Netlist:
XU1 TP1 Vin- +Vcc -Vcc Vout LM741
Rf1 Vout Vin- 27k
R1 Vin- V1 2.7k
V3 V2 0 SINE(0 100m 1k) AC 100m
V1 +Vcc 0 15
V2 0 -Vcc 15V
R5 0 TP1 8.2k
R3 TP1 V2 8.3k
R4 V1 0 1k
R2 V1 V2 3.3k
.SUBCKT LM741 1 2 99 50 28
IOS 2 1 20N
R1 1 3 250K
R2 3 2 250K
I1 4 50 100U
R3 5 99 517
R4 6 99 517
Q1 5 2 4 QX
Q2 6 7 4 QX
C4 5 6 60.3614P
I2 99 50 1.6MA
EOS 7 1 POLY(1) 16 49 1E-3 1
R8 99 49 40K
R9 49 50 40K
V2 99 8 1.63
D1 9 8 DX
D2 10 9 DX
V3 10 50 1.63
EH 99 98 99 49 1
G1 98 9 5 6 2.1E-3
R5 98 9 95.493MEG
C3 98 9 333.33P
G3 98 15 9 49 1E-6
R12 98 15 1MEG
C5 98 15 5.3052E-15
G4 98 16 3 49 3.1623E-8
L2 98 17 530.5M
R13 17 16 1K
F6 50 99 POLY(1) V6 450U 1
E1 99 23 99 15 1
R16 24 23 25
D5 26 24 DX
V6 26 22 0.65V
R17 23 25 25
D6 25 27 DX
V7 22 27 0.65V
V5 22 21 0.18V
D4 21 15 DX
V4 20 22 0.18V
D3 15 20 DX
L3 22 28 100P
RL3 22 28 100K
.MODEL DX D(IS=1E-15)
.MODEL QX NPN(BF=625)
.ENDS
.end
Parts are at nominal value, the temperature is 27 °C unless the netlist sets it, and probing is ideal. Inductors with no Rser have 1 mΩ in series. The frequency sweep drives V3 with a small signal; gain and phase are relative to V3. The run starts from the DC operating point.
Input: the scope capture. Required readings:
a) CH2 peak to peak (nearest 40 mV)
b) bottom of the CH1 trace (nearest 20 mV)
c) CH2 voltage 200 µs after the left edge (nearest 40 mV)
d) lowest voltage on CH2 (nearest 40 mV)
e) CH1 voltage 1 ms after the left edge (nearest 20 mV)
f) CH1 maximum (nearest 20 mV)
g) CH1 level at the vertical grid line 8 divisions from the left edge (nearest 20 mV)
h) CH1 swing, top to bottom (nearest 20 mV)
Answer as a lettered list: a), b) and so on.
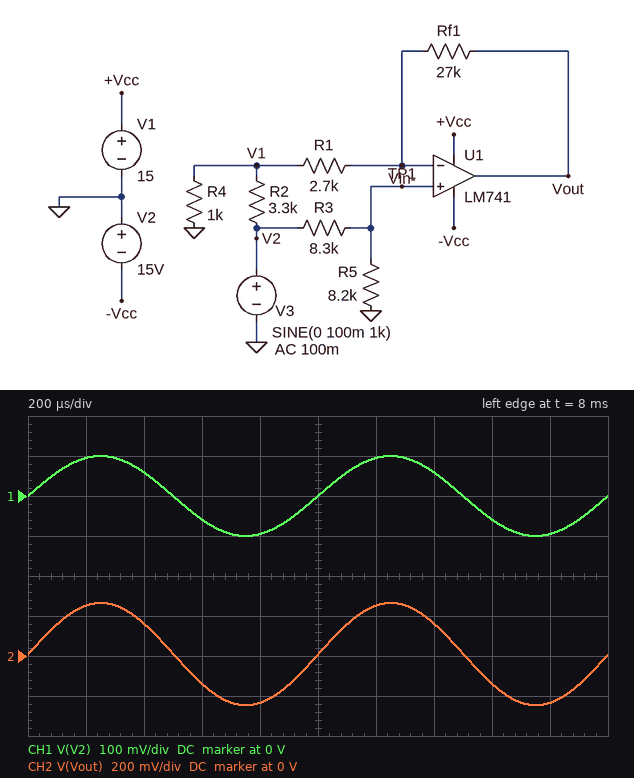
a) 520 mV
b) -100 mV
c) 240 mV
d) -240 mV
e) 0 V
f) 100 mV
g) -60 mV
h) 200 mV
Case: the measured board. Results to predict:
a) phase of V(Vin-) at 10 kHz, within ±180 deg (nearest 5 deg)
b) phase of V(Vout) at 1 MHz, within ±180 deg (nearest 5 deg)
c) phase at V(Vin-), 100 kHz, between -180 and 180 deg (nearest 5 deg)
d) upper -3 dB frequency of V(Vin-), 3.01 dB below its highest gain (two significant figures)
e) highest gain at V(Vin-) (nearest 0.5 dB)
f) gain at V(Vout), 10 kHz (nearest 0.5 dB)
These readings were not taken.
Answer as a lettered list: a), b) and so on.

a) -5 deg
b) -100 deg
c) -20 deg
d) 140 kHz
e) -6.0 dB
f) 8.0 dB
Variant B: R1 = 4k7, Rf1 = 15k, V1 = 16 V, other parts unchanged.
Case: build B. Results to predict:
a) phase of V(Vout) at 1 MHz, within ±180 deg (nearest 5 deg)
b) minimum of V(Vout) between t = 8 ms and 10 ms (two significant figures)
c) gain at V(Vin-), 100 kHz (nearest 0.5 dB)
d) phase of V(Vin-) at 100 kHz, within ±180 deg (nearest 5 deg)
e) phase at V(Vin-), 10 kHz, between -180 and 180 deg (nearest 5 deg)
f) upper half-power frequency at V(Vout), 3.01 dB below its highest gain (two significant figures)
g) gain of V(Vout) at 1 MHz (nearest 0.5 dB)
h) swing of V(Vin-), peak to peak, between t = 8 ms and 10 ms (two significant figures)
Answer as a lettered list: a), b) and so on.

a) -95 deg
b) -120 mV
c) -6.5 dB
d) -15 deg
e) 0 deg
f) 290 kHz
g) -10.0 dB
h) 99 mV
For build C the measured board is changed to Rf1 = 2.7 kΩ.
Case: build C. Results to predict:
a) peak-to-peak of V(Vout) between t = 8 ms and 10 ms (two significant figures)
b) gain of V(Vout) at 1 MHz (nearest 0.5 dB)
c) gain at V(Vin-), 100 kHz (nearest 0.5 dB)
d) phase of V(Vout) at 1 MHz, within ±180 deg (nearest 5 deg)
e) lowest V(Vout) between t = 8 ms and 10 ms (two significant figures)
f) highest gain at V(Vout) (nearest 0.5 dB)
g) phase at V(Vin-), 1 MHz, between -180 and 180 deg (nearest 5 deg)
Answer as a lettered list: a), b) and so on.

a) 140 mV
b) -8.0 dB
c) -6.0 dB
d) -80 deg
e) -69 mV
f) -3.0 dB
g) -55 deg
